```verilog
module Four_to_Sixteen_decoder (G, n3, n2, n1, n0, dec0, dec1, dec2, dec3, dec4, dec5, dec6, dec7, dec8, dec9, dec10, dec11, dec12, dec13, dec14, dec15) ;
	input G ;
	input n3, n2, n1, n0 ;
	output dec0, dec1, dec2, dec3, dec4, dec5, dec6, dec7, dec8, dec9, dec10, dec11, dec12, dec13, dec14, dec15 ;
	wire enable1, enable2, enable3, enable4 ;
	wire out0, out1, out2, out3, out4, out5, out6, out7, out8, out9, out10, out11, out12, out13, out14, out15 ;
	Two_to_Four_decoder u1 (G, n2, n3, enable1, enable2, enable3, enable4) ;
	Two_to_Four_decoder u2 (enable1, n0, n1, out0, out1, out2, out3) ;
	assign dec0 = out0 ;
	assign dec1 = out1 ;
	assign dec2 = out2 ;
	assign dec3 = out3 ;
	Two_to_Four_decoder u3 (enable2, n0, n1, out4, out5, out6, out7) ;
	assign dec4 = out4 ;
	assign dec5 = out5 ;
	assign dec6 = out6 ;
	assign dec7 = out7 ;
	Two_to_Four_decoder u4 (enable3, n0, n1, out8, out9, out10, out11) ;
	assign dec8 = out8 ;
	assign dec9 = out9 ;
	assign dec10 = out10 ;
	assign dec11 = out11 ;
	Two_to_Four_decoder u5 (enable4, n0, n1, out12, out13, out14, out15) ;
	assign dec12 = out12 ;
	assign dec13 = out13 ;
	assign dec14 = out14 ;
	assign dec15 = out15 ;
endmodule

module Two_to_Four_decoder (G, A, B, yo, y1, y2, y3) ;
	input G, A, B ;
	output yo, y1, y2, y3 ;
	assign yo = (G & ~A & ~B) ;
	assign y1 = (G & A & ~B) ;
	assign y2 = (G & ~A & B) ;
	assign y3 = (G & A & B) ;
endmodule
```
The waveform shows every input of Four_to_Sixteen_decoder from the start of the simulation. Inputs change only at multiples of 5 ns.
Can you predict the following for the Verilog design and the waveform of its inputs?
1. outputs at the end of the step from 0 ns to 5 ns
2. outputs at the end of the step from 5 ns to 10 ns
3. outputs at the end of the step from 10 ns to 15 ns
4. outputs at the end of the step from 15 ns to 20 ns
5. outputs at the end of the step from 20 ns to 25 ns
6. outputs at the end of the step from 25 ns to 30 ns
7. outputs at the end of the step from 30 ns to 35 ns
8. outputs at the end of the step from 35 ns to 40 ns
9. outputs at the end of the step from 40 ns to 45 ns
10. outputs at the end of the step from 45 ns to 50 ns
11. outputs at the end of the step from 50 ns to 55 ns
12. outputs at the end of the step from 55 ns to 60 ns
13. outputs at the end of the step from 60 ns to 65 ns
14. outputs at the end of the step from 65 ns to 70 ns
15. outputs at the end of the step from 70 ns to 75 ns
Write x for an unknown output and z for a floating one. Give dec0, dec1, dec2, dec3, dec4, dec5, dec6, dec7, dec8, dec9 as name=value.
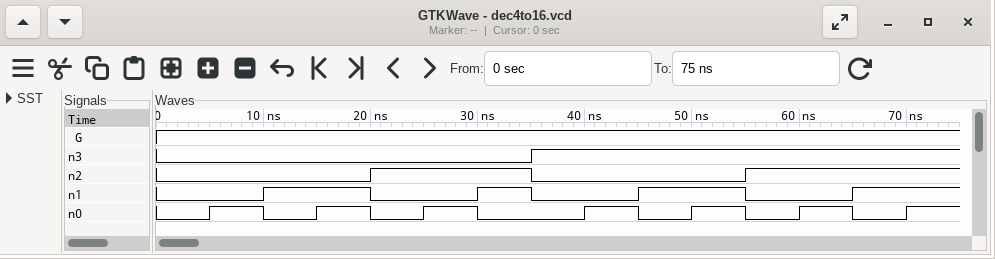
dec0=1, dec1=0, dec2=0, dec3=0, dec4=0, dec5=0, dec6=0, dec7=0, dec8=0, dec9=0
dec0=0, dec1=1, dec2=0, dec3=0, dec4=0, dec5=0, dec6=0, dec7=0, dec8=0, dec9=0
dec0=0, dec1=0, dec2=1, dec3=0, dec4=0, dec5=0, dec6=0, dec7=0, dec8=0, dec9=0
dec0=0, dec1=0, dec2=0, dec3=1, dec4=0, dec5=0, dec6=0, dec7=0, dec8=0, dec9=0
dec0=0, dec1=0, dec2=0, dec3=0, dec4=1, dec5=0, dec6=0, dec7=0, dec8=0, dec9=0
dec0=0, dec1=0, dec2=0, dec3=0, dec4=0, dec5=1, dec6=0, dec7=0, dec8=0, dec9=0
dec0=0, dec1=0, dec2=0, dec3=0, dec4=0, dec5=0, dec6=1, dec7=0, dec8=0, dec9=0
dec0=0, dec1=0, dec2=0, dec3=0, dec4=0, dec5=0, dec6=0, dec7=0, dec8=1, dec9=0
dec0=0, dec1=0, dec2=0, dec3=0, dec4=0, dec5=0, dec6=0, dec7=0, dec8=0, dec9=1
dec0=0, dec1=0, dec2=0, dec3=0, dec4=0, dec5=0, dec6=0, dec7=0, dec8=0, dec9=0
dec0=0, dec1=0, dec2=0, dec3=0, dec4=0, dec5=0, dec6=0, dec7=0, dec8=0, dec9=0
dec0=0, dec1=0, dec2=0, dec3=0, dec4=0, dec5=0, dec6=0, dec7=0, dec8=0, dec9=0
dec0=0, dec1=0, dec2=0, dec3=0, dec4=0, dec5=0, dec6=0, dec7=0, dec8=0, dec9=0
dec0=0, dec1=0, dec2=0, dec3=0, dec4=0, dec5=0, dec6=0, dec7=0, dec8=0, dec9=0
dec0=0, dec1=0, dec2=0, dec3=0, dec4=0, dec5=0, dec6=0, dec7=0, dec8=0, dec9=0
